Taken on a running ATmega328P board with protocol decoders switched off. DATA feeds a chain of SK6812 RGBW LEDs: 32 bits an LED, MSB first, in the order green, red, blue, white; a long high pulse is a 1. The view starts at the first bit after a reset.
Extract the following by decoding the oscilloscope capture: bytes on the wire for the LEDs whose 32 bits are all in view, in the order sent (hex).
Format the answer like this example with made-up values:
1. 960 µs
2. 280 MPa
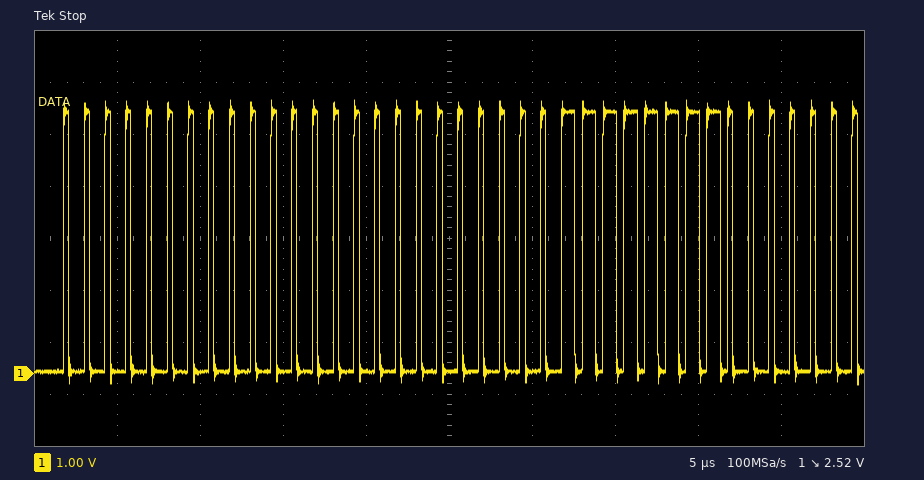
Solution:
1. 00 00 00 FF
